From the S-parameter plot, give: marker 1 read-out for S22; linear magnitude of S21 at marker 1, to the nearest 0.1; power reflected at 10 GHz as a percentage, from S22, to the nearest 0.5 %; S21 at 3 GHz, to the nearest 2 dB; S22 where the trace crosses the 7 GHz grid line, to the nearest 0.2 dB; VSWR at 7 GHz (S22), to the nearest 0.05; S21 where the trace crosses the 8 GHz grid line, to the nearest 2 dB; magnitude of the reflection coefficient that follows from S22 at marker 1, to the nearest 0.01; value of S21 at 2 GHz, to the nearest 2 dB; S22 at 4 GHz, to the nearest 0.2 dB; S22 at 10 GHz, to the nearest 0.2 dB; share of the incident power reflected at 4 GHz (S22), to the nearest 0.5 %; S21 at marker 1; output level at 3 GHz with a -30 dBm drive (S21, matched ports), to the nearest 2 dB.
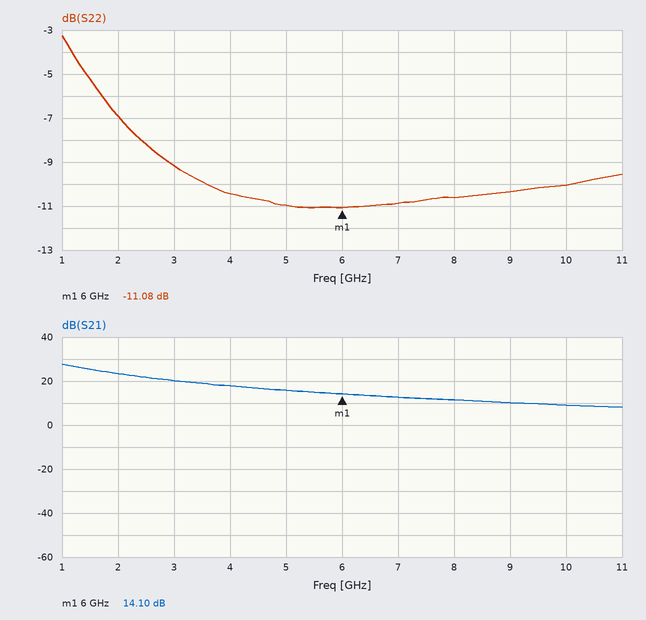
-11.08 dB
5.1
10.0 %
20 dB
-10.8 dB
1.80
12 dB
0.28
24 dB
-10.4 dB
-10.0 dB
9.0 %
14.10 dB
-10 dBm
